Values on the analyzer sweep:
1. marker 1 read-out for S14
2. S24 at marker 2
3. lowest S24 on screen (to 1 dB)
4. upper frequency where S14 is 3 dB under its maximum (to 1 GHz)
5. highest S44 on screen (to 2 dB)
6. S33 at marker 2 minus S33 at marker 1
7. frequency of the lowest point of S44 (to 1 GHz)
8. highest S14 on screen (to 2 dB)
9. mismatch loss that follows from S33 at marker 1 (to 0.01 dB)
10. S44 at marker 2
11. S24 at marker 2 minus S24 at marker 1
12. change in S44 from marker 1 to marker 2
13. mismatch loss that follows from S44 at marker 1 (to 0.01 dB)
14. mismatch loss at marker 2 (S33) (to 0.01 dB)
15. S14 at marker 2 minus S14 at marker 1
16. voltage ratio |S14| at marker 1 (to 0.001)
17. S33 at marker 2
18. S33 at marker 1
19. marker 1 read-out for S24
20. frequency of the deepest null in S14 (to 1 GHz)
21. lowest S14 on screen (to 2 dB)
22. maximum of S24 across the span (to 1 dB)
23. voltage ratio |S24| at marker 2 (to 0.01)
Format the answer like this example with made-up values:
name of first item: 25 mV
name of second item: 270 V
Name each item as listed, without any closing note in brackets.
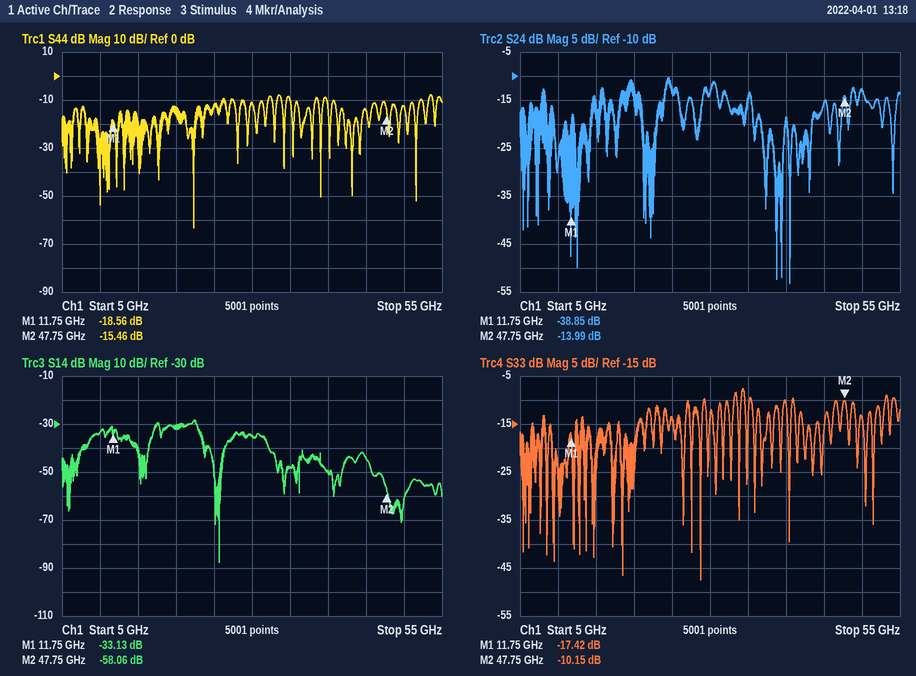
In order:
marker 1 read-out for S14: -33.13 dB
S24 at marker 2: -13.99 dB
lowest S24 on screen: -53 dB
upper frequency where S14 is 3 dB under its maximum: 23 GHz
highest S44 on screen: -8 dB
S33 at marker 2 minus S33 at marker 1: 7.27 dB
frequency of the lowest point of S44: 22 GHz
highest S14 on screen: -28 dB
mismatch loss that follows from S33 at marker 1: 0.08 dB
S44 at marker 2: -15.46 dB
S24 at marker 2 minus S24 at marker 1: 24.86 dB
change in S44 from marker 1 to marker 2: 3.10 dB
mismatch loss that follows from S44 at marker 1: 0.06 dB
mismatch loss at marker 2 (S33): 0.44 dB
S14 at marker 2 minus S14 at marker 1: -24.93 dB
voltage ratio |S14| at marker 1: 0.022
S33 at marker 2: -10.15 dB
S33 at marker 1: -17.42 dB
marker 1 read-out for S24: -38.85 dB
frequency of the deepest null in S14: 26 GHz
lowest S14 on screen: -88 dB
maximum of S24 across the span: -10 dB
voltage ratio |S24| at marker 2: 0.20
